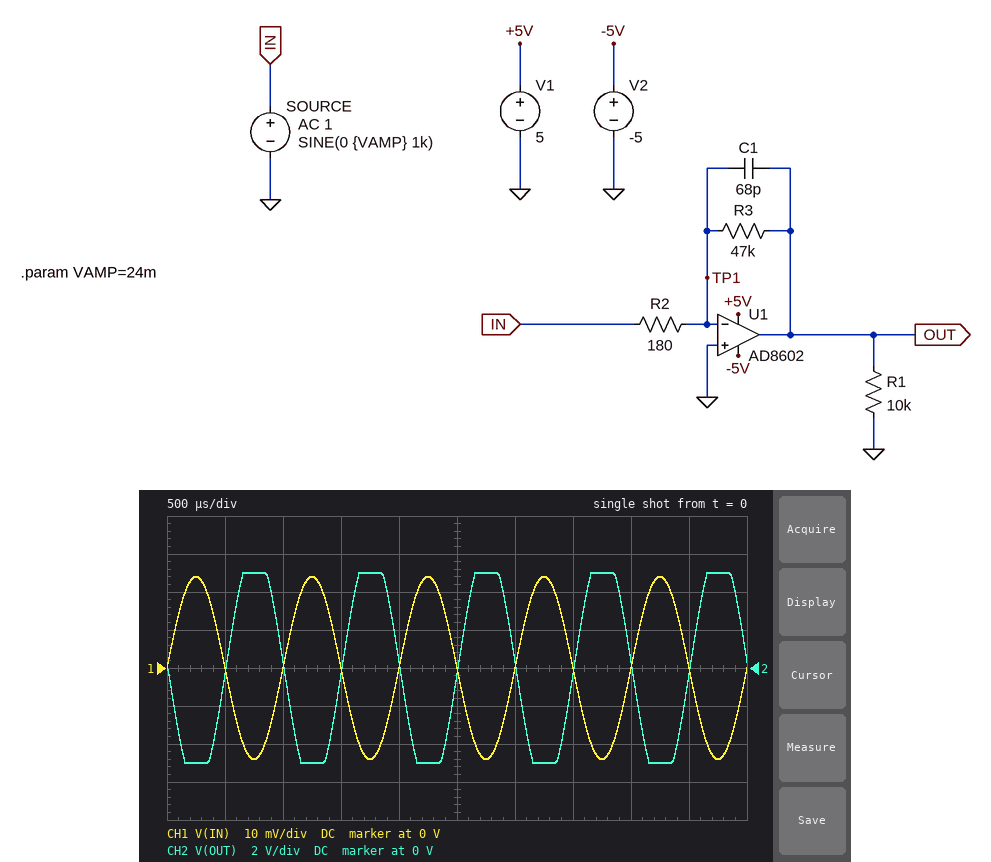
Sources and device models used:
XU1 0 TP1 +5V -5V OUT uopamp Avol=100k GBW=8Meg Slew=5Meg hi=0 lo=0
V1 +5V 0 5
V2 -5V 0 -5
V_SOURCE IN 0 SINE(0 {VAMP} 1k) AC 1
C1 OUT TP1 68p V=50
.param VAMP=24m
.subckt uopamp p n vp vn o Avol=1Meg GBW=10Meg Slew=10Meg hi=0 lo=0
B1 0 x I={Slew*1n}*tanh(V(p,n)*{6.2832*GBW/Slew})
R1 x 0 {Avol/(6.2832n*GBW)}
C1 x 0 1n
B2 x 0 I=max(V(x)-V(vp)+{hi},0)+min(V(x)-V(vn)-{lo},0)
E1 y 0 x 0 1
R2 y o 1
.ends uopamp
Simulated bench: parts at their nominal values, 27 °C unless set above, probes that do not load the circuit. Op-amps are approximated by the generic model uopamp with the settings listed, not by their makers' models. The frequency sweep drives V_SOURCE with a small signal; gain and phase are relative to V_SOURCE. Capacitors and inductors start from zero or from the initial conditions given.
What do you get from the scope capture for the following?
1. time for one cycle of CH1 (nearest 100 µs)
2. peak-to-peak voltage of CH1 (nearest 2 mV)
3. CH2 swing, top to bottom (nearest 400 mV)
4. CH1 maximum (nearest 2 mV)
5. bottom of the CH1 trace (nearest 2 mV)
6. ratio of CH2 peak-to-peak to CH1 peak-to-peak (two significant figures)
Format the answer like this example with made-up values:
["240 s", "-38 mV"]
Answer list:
["1.0 ms", "48 mV", "10.0 V", "24 mV", "-24 mV", "210"]
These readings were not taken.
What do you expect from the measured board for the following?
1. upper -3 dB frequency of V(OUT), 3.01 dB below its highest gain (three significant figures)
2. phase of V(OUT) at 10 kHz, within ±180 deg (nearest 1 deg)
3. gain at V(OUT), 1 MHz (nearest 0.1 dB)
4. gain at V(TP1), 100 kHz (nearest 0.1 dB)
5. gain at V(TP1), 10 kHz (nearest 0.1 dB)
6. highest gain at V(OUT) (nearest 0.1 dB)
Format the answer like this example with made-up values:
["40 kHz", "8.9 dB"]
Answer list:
["19.0 kHz", "152 deg", "13.9 dB", "-4.3 dB", "-10.8 dB", "48.3 dB"]
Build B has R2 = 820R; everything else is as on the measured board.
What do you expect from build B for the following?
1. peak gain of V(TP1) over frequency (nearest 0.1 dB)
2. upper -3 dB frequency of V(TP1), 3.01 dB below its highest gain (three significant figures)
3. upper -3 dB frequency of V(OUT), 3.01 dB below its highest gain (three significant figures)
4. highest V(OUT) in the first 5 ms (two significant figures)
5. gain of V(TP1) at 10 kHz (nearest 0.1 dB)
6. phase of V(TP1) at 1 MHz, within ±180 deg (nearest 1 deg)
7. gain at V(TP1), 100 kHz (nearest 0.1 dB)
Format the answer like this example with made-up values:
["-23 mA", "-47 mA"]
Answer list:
["-11.6 dB", "10.9 MHz", "36.7 kHz", "1.4 V", "-23.2 dB", "-3 deg", "-12.2 dB"]
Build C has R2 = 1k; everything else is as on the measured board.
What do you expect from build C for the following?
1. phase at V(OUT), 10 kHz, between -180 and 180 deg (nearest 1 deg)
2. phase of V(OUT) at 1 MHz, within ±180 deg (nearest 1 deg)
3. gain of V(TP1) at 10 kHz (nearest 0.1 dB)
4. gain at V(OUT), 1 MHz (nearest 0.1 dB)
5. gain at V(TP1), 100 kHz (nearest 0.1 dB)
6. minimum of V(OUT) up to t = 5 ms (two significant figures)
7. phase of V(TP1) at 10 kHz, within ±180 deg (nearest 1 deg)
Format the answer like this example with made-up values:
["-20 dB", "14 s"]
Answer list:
["165 deg", "87 deg", "-24.9 dB", "5.1 dB", "-13.5 dB", "-1.1 V", "75 deg"]
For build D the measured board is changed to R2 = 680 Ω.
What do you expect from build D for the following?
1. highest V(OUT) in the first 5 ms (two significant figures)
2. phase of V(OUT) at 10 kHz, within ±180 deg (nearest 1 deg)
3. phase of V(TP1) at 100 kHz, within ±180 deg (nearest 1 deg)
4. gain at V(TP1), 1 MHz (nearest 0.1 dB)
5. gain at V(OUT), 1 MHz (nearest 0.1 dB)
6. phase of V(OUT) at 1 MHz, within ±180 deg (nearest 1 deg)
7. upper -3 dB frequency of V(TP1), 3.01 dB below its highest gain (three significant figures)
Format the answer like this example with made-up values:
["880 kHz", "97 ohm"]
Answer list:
["1.7 V", "164 deg", "19 deg", "-10.5 dB", "7.6 dB", "87 deg", "11.5 MHz"]
